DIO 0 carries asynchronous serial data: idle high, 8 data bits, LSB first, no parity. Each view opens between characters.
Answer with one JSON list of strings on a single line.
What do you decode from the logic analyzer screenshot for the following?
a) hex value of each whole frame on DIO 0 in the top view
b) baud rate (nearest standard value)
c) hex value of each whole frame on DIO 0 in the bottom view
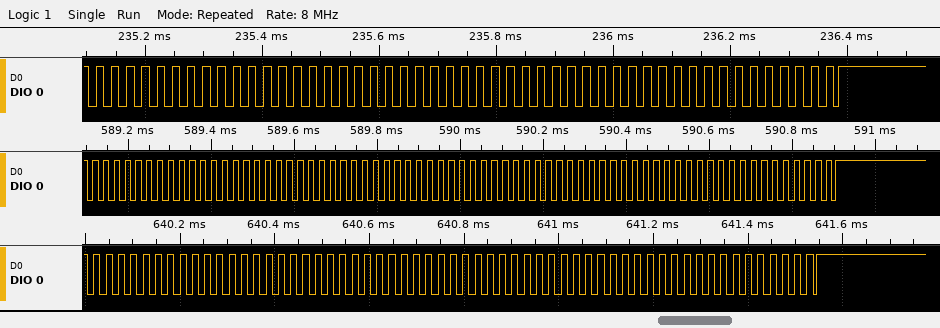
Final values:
["55, 55, 55, 55, 55, 55, 55, 55, 55, D5", "74880 baud", "55, 55, 55, 55, 55, 55, 55, 55, 55, 55, 55, D5"]
